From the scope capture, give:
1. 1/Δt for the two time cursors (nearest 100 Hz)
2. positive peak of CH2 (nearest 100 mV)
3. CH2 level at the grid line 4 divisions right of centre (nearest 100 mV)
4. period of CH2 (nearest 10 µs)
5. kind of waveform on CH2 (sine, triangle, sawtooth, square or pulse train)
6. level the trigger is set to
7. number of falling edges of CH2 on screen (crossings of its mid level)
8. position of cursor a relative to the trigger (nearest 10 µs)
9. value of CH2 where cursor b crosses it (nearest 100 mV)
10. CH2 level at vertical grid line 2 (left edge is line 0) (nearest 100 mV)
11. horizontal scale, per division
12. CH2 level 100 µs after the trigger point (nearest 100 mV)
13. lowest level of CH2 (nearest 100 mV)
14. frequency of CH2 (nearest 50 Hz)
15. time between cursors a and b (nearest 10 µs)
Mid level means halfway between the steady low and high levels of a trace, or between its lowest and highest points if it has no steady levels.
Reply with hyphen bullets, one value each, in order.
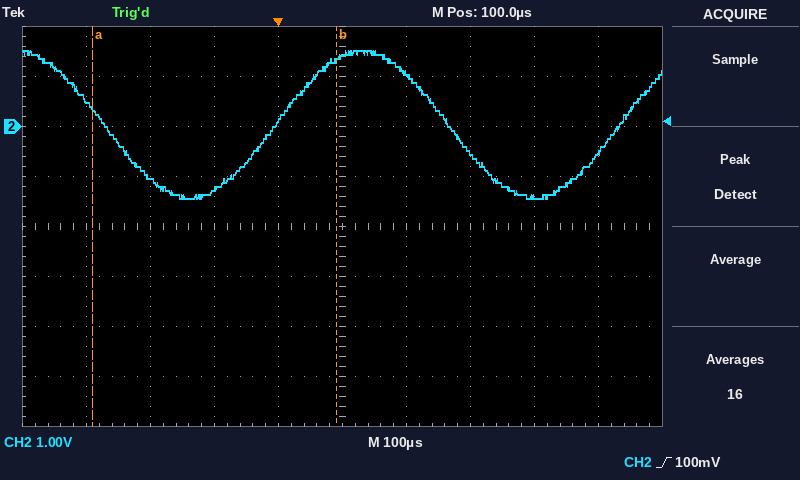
- 2.6 kHz
- 1.5 V
- -500 mV
- 540 µs
- sine
- 100 mV
- 2
- -290 µs
- 1.4 V
- -1.0 V
- 100 µs
- 1.4 V
- -1.4 V
- 1.85 kHz
- 380 µs
